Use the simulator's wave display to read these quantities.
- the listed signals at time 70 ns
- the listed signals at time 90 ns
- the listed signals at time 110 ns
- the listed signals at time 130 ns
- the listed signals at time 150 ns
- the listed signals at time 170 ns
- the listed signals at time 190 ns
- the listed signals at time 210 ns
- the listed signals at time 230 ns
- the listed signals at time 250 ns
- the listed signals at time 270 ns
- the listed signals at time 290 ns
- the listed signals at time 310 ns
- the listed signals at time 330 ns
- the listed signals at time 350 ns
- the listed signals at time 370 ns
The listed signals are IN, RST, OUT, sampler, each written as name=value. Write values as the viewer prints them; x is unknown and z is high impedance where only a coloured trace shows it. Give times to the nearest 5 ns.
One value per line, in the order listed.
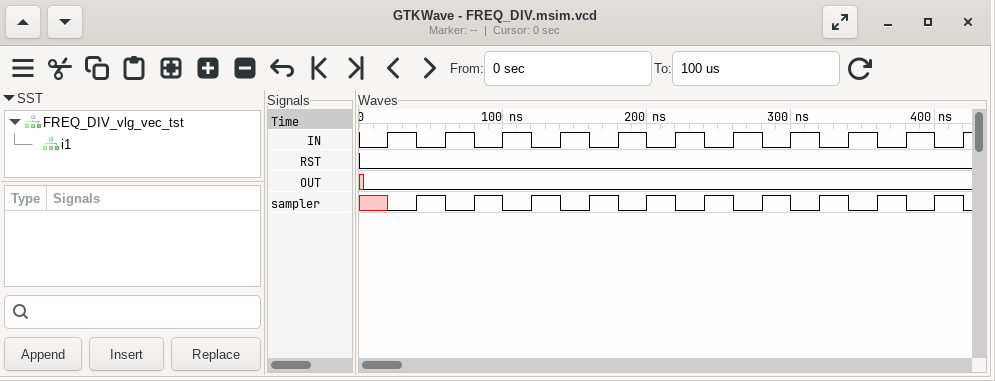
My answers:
IN=1, RST=0, OUT=0, sampler=0
IN=0, RST=0, OUT=0, sampler=1
IN=1, RST=0, OUT=0, sampler=0
IN=0, RST=0, OUT=0, sampler=1
IN=1, RST=0, OUT=0, sampler=0
IN=0, RST=0, OUT=0, sampler=1
IN=1, RST=0, OUT=0, sampler=0
IN=0, RST=0, OUT=0, sampler=1
IN=1, RST=0, OUT=0, sampler=0
IN=0, RST=0, OUT=0, sampler=1
IN=1, RST=0, OUT=0, sampler=0
IN=0, RST=0, OUT=0, sampler=1
IN=1, RST=0, OUT=0, sampler=0
IN=0, RST=0, OUT=0, sampler=1
IN=1, RST=0, OUT=0, sampler=0
IN=0, RST=0, OUT=0, sampler=1
